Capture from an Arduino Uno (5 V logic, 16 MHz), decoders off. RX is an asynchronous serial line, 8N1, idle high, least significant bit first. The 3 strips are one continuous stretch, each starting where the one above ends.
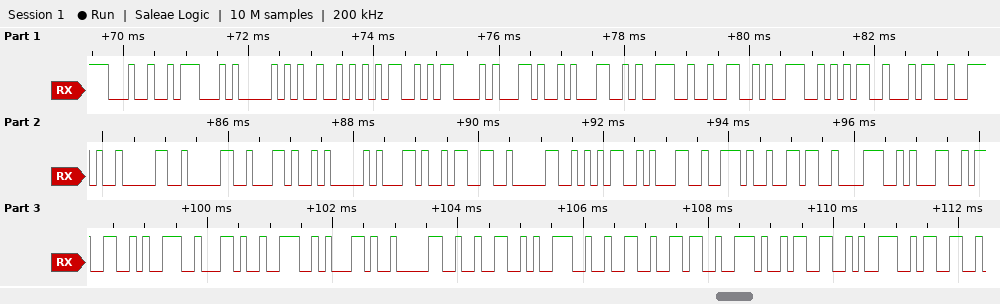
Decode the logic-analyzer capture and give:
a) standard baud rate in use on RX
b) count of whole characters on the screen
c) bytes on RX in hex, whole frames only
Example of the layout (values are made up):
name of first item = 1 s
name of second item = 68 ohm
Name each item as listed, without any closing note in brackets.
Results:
standard baud rate in use on RX = 9600 baud
count of whole characters on the screen = 41
bytes on RX in hex, whole frames only = 24 47 50 52 4D 43 2C 31 39 32 39 35 34 2E 30 30 2C 41 2C 33 30 35 31 2E 36 38 31 33 39 2C 4E 2C 30 32 39 32 36 2E 33 39 33
